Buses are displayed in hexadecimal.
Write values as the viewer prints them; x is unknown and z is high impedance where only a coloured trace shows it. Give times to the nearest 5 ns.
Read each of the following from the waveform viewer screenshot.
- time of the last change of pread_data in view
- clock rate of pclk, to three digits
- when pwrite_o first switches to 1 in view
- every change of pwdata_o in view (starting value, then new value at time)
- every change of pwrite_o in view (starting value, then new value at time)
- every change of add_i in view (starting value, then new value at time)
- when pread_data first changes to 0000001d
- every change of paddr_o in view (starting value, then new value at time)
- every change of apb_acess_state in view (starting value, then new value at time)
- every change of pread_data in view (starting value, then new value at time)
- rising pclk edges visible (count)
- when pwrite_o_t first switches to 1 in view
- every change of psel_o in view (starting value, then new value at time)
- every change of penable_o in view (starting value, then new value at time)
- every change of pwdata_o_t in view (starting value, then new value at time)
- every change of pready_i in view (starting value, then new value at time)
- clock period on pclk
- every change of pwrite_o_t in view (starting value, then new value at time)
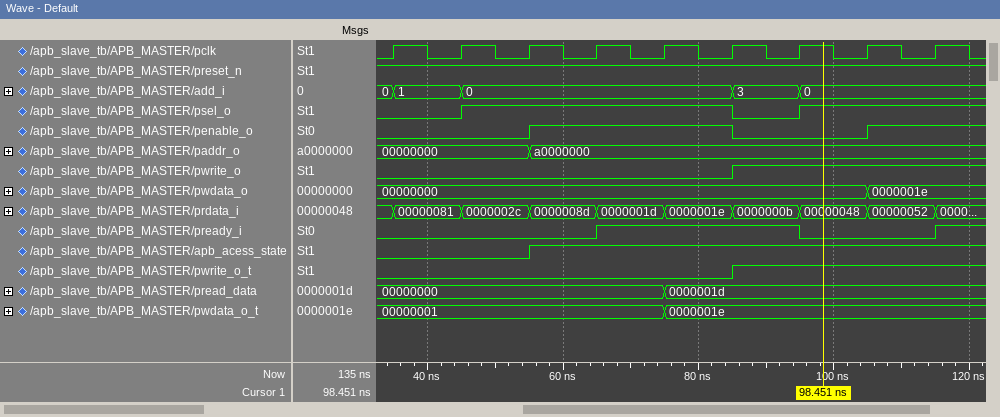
75 ns
100 MHz
85 ns
00000000, 0000001e at 105 ns
0, 1 at 85 ns
0, 1 at 35 ns, 0 at 45 ns, 3 at 85 ns, 0 at 95 ns
75 ns
00000000, a0000000 at 55 ns
0, 1 at 55 ns
00000000, 0000001d at 75 ns
9
85 ns
0, 1 at 45 ns, 0 at 85 ns, 1 at 95 ns
0, 1 at 55 ns, 0 at 85 ns, 1 at 105 ns
00000001, 0000001e at 75 ns
0, 1 at 65 ns, 0 at 95 ns, 1 at 115 ns
10 ns
0, 1 at 85 ns
